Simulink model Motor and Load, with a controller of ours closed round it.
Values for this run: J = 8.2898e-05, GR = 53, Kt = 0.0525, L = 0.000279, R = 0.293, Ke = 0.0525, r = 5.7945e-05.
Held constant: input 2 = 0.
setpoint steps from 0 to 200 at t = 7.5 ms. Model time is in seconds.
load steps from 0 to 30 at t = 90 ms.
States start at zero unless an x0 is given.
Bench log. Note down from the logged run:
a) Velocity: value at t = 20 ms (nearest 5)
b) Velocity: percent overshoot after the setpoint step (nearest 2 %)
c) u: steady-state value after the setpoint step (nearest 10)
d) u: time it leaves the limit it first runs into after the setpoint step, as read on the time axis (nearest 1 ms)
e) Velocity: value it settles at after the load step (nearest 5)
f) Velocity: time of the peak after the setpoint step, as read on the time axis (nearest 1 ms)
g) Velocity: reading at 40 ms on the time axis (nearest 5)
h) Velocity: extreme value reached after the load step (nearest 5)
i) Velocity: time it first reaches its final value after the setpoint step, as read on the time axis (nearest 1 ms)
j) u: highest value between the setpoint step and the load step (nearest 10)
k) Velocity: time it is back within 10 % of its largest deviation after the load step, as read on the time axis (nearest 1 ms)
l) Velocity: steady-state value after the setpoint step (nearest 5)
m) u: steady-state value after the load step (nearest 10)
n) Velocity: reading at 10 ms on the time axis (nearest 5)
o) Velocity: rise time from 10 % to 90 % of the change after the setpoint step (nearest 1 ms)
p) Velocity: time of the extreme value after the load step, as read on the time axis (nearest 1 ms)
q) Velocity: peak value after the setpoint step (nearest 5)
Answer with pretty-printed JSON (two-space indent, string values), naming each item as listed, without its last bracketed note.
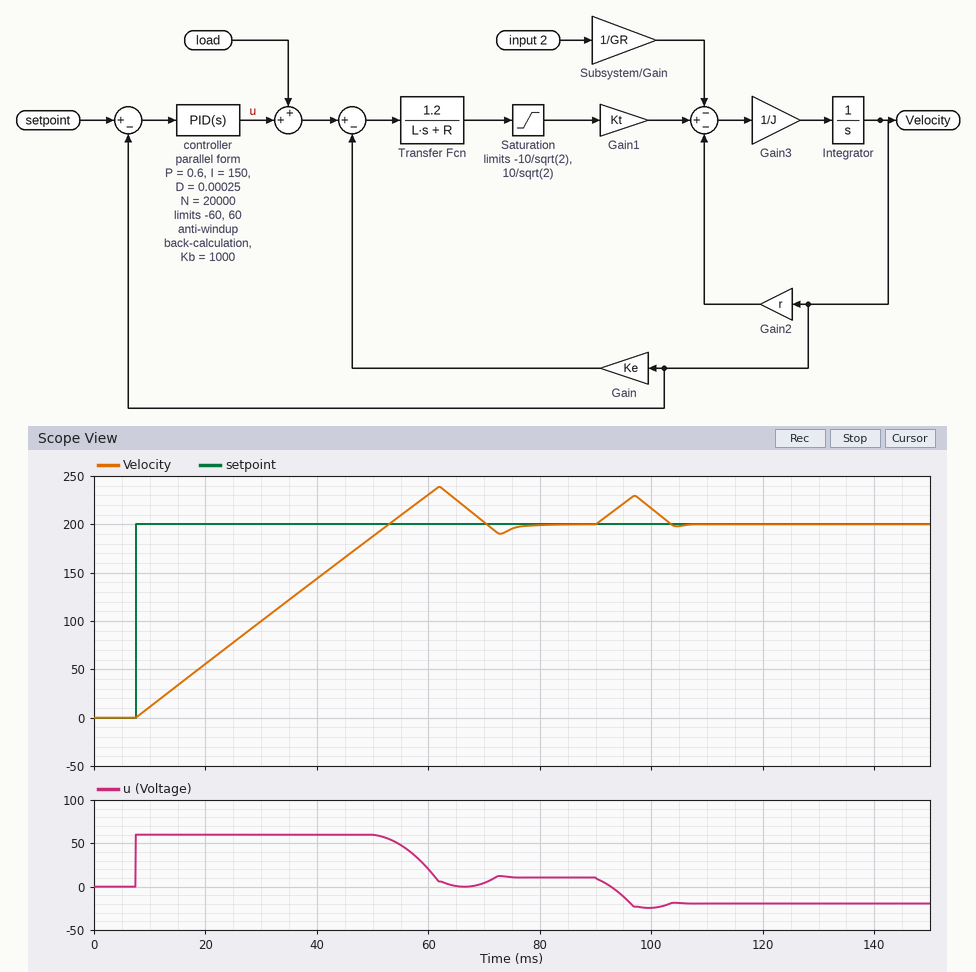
{
  "Velocity: value at t = 20 ms": "55",
  "Velocity: percent overshoot after the setpoint step": "20 %",
  "u: steady-state value after the setpoint step": "10",
  "u: time it leaves the limit it first runs into after the setpoint step, as read on the time axis": "51 ms",
  "Velocity: value it settles at after the load step": "200",
  "Velocity: time of the peak after the setpoint step, as read on the time axis": "62 ms",
  "Velocity: reading at 40 ms on the time axis": "145",
  "Velocity: extreme value reached after the load step": "230",
  "Velocity: time it first reaches its final value after the setpoint step, as read on the time axis": "53 ms",
  "u: highest value between the setpoint step and the load step": "60",
  "Velocity: time it is back within 10 % of its largest deviation after the load step, as read on the time axis": "103 ms",
  "Velocity: steady-state value after the setpoint step": "200",
  "u: steady-state value after the load step": "-20",
  "Velocity: reading at 10 ms on the time axis": "10",
  "Velocity: rise time from 10 % to 90 % of the change after the setpoint step": "36 ms",
  "Velocity: time of the extreme value after the load step, as read on the time axis": "97 ms",
  "Velocity: peak value after the setpoint step": "240"
}
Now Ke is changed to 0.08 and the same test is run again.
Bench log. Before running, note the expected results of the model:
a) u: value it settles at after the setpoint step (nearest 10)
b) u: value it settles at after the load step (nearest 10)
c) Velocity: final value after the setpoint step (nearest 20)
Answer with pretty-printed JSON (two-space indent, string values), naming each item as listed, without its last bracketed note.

{
  "u: value it settles at after the setpoint step": "20",
  "u: value it settles at after the load step": "-10",
  "Velocity: final value after the setpoint step": "200"
}
